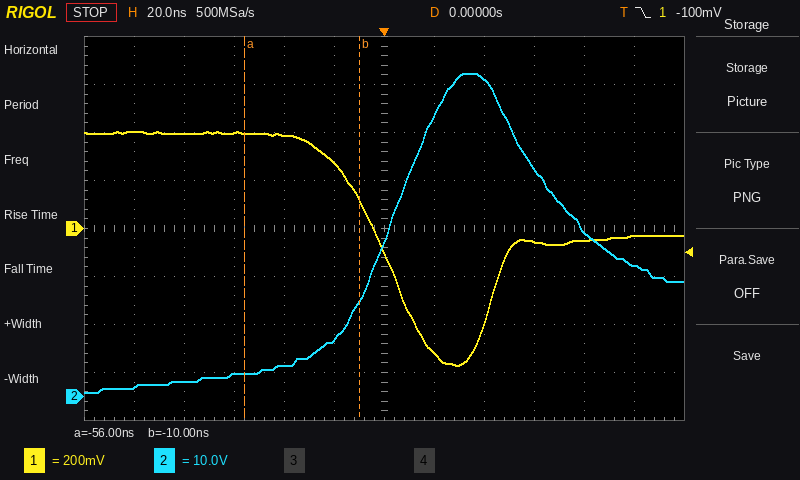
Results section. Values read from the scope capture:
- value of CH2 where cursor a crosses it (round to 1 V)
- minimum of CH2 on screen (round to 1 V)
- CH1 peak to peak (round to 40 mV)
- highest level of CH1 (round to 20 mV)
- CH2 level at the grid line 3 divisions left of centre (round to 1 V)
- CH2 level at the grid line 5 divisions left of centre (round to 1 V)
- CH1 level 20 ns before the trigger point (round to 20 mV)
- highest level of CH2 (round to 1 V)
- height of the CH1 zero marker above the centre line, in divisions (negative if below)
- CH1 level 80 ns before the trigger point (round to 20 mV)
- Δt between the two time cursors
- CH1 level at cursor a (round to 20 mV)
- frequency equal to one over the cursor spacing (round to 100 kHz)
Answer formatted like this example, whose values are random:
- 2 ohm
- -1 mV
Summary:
- 5 V
- 1 V
- 960 mV
- 400 mV
- 5 V
- 2 V
- 280 mV
- 67 V
- 0.0 div
- 400 mV
- 46 ns
- 400 mV
- 21.7 MHz
